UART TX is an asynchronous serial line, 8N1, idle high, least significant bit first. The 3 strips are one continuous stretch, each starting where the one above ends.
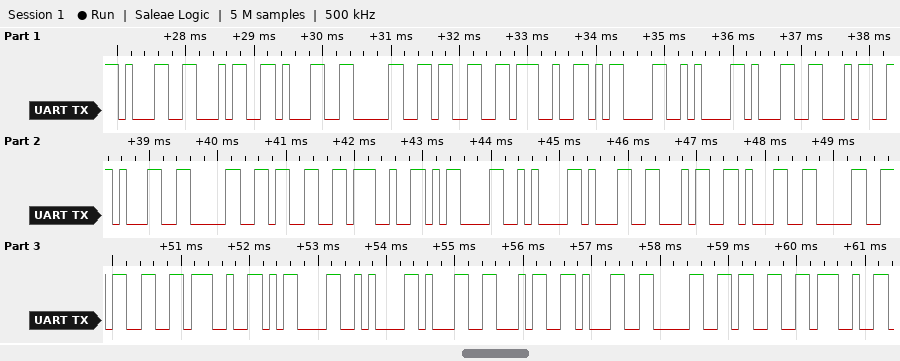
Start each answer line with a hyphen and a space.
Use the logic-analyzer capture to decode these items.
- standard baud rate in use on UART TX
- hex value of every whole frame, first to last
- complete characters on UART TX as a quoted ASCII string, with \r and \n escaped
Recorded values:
- 9600 baud
- 0x31 0x34 0x31 0x30 0x33 0x27 0x0D 0x0A 0x31 0x34 0x31 0x30 0x33 0x27 0x0D 0x0A 0x31 0x34 0x31 0x30 0x33 0x27 0x0D 0x0A 0x31 0x34 0x31 0x30 0x33 0x27
- "14103'\r\n14103'\r\n14103'\r\n14103'"
